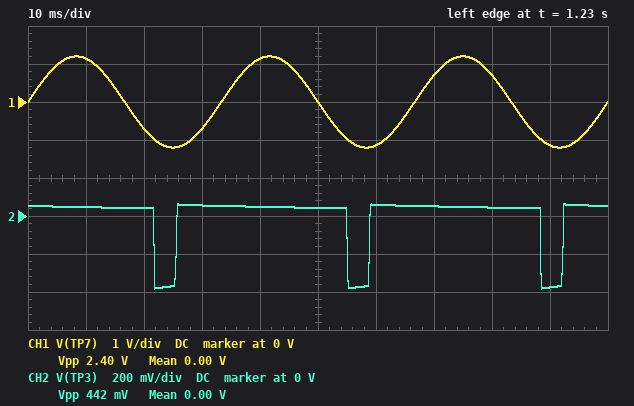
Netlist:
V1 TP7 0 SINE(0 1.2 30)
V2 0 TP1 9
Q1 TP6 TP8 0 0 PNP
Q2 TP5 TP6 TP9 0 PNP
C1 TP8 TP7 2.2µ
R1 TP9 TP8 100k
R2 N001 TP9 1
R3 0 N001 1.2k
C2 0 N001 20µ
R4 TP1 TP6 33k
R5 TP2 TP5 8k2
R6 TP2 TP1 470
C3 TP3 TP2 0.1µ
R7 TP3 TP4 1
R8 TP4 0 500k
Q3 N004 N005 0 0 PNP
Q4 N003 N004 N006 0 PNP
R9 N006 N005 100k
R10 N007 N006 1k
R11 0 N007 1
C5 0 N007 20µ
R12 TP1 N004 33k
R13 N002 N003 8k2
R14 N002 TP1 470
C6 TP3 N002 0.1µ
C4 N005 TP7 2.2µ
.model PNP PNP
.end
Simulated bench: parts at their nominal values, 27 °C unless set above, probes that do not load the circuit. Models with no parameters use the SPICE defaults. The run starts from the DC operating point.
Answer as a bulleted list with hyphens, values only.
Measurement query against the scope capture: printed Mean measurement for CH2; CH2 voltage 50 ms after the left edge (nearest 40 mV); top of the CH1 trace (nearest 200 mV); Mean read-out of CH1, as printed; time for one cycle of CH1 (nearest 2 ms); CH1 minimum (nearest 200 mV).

- 0.00 V
- 40 mV
- 1.2 V
- 0.00 V
- 34 ms
- -1.2 V
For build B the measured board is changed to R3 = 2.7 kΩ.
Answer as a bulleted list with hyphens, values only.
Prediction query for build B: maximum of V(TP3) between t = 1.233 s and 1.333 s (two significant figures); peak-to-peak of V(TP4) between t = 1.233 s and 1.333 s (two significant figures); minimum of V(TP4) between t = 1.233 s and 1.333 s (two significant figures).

- 63 mV
- 410 mV
- -350 mV
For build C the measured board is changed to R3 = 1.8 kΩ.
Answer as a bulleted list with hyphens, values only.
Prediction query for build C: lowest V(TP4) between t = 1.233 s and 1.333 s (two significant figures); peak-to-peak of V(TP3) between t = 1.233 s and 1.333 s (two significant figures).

- -370 mV
- 430 mV
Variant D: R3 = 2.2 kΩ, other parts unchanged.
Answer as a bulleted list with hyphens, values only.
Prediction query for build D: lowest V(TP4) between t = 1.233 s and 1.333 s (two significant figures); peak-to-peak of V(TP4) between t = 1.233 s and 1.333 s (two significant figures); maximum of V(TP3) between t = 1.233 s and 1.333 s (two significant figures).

- -360 mV
- 420 mV
- 63 mV
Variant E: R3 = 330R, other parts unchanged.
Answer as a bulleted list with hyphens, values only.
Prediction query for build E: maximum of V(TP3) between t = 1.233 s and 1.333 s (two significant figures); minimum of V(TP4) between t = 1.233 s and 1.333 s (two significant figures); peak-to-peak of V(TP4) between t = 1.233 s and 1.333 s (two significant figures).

- 56 mV
- -410 mV
- 460 mV
